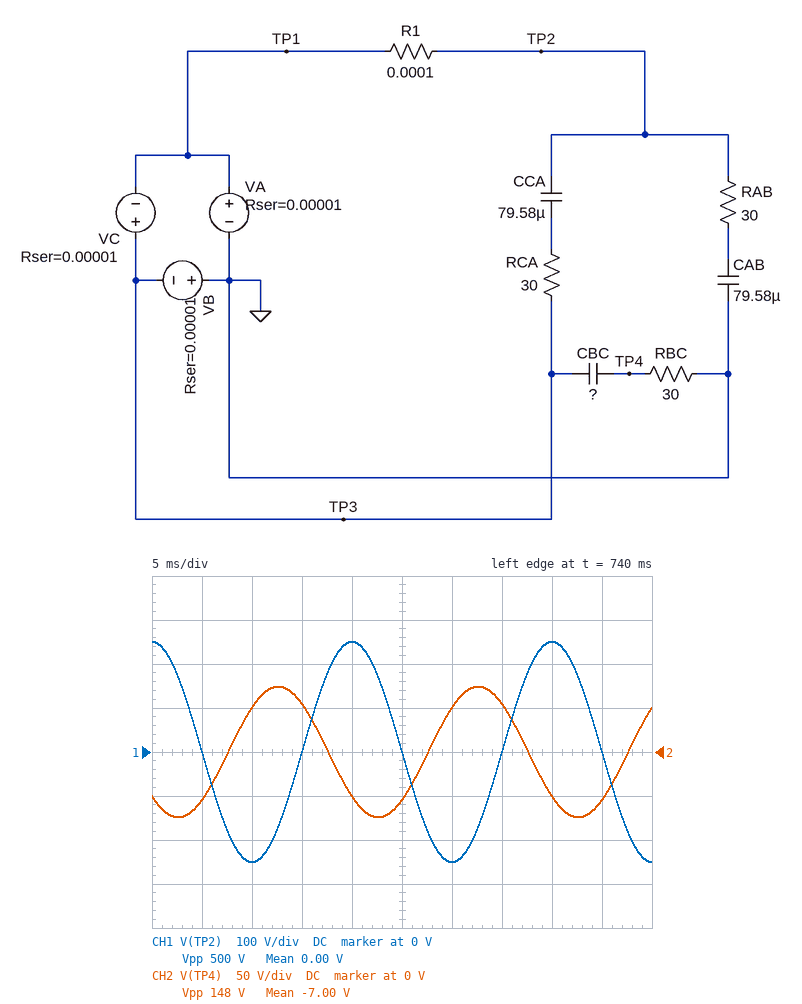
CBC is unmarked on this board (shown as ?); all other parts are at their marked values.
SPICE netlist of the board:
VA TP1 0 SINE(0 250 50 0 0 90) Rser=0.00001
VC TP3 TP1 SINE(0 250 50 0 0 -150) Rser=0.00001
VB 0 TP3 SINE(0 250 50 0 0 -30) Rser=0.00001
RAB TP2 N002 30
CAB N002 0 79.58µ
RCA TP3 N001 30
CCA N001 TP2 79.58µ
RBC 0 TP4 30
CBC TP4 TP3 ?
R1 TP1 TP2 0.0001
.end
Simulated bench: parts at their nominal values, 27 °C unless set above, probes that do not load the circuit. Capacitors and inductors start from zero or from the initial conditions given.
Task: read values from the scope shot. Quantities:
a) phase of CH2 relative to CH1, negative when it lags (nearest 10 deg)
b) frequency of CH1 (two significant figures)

130 deg
50 Hz
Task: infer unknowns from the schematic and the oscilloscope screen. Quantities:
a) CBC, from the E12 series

33 µF
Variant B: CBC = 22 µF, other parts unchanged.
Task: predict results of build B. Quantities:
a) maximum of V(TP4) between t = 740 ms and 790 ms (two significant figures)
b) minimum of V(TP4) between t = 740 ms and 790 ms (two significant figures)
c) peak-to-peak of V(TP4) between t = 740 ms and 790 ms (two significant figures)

51 V
-51 V
100 V
